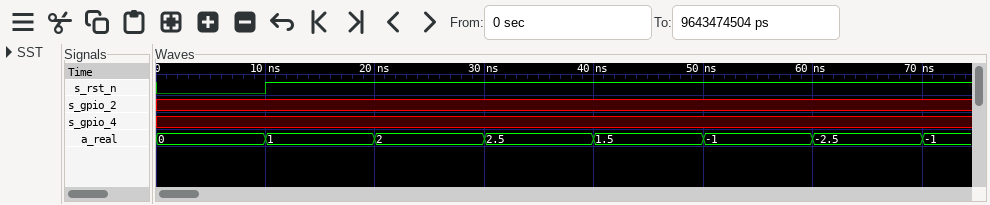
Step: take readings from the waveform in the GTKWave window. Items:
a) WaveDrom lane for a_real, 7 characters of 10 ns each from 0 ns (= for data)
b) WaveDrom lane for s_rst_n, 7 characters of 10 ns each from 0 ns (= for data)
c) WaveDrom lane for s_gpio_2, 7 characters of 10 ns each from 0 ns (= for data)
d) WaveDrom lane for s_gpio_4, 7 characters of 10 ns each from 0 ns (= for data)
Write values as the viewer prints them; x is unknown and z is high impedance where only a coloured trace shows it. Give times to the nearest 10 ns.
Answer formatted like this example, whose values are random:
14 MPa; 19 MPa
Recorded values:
{name: 'a_real', wave: '=======', data: '0 1 2 2.5 1.5 -1 -2.5'}; {name: 's_rst_n', wave: '01.....'}; {name: 's_gpio_2', wave: 'x......'}; {name: 's_gpio_4', wave: 'x......'}
